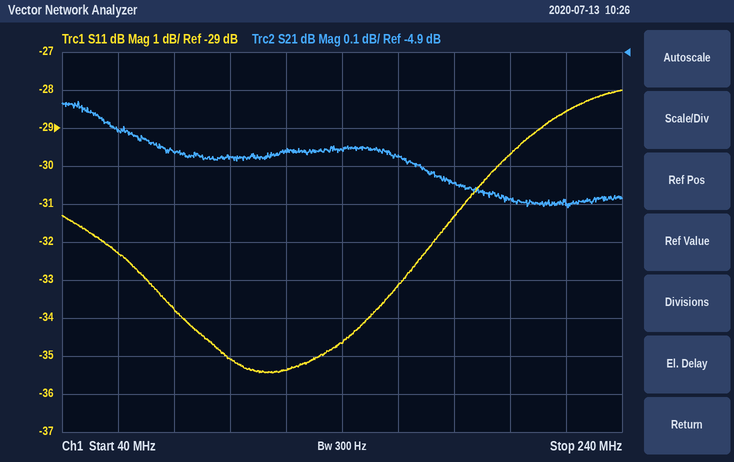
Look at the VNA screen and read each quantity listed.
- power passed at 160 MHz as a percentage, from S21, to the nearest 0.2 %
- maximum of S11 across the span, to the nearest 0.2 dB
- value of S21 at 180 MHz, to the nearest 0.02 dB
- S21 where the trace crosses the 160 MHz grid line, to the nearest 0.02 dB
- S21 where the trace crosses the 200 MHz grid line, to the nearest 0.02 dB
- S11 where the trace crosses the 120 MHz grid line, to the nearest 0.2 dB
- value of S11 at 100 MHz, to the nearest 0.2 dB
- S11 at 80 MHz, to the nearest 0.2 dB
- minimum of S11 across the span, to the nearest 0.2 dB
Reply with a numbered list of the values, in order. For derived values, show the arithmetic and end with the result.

1. 10^(-5.18/10) ≈ 30.3 %, so 30.4 % to the nearest 0.2 %
2. -28.0 dB
3. -5.24 dB
4. -5.18 dB
5. -5.28 dB
6. -35.4 dB
7. -35.0 dB
8. -33.8 dB
9. -35.4 dB
